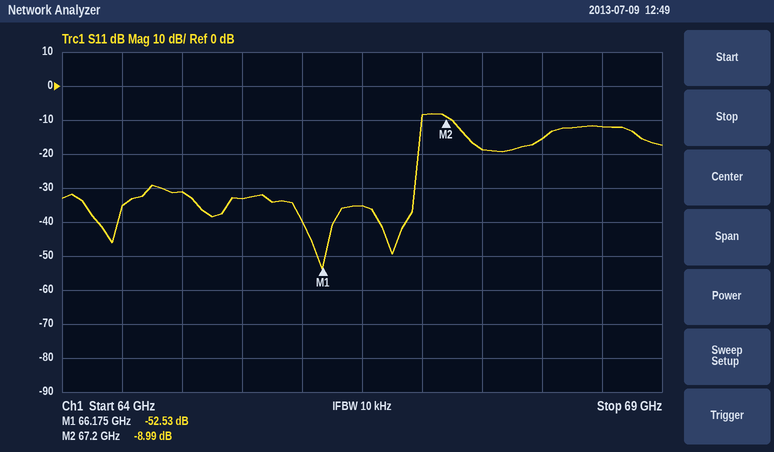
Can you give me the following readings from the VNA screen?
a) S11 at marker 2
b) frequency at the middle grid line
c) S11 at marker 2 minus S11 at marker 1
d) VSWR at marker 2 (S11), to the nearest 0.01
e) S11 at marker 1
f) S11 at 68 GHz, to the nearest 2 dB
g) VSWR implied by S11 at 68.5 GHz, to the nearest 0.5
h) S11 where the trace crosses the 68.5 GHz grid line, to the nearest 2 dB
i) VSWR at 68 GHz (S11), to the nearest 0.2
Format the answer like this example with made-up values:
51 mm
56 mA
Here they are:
-8.99 dB
66.5 GHz
43.54 dB
2.10
-52.53 dB
-16 dB
1.5
-12 dB
1.4
